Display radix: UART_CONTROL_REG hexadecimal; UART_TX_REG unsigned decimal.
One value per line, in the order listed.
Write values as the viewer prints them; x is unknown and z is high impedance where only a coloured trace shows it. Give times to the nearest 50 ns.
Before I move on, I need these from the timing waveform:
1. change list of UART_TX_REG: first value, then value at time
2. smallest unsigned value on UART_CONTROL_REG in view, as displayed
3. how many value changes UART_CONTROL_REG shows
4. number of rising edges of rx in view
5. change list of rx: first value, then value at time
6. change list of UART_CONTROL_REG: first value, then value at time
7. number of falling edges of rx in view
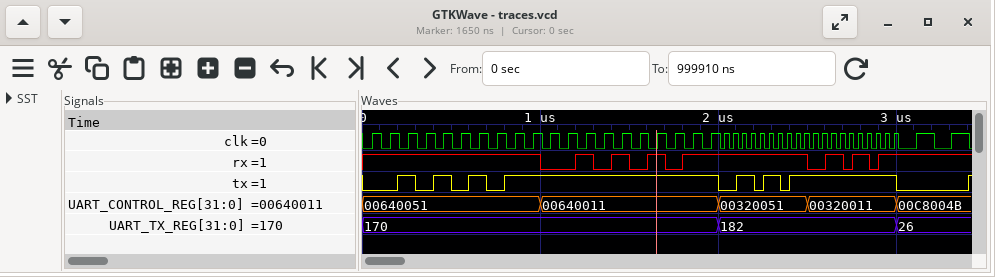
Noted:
170, 182 at 2000 ns, 26 at 3000 ns
00320011
4
7
1, 0 at 1000 ns, 1 at 1200 ns, 0 at 1300 ns, 1 at 1400 ns, 0 at 1500 ns, 1 at 1600 ns, 0 at 1700 ns, 1 at 1800 ns, 0 at 2500 ns, 1 at 2600 ns, 0 at 2700 ns, 1 at 2750 ns, 0 at 2850 ns, 1 at 2900 ns
00640051, 00640011 at 1000 ns, 00320051 at 2000 ns, 00320011 at 2500 ns, 00C8004B at 3000 ns
7
